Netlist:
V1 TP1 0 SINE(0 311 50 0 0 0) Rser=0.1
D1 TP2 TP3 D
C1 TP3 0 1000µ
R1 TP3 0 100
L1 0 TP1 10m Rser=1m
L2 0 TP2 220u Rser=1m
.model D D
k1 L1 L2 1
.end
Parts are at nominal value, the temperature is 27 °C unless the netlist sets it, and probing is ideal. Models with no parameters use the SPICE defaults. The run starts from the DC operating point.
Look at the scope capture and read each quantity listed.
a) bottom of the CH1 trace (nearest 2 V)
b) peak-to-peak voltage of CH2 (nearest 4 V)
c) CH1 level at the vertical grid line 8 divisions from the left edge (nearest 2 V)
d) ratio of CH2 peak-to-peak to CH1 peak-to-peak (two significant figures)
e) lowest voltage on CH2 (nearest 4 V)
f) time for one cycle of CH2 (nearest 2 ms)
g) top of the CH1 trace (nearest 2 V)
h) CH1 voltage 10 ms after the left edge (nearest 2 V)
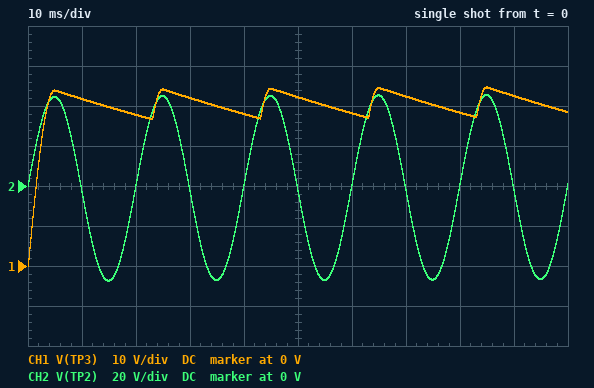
0 V
92 V
38 V
2.1
-48 V
20 ms
44 V
42 V
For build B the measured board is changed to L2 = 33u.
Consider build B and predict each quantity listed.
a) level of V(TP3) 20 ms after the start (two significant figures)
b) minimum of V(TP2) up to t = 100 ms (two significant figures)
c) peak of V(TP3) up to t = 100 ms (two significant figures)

14 V
-18 V
17 V
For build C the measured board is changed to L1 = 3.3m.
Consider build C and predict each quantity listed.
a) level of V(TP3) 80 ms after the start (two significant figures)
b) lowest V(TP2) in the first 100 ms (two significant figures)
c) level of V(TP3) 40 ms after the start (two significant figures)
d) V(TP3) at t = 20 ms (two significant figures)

67 V
-85 V
65 V
62 V
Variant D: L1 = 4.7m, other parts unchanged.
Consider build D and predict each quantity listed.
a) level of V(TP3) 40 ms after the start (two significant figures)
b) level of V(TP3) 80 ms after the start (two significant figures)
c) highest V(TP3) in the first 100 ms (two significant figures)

55 V
56 V
66 V
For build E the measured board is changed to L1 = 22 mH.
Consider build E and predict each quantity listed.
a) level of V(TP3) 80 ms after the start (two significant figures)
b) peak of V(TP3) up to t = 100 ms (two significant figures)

26 V
30 V
